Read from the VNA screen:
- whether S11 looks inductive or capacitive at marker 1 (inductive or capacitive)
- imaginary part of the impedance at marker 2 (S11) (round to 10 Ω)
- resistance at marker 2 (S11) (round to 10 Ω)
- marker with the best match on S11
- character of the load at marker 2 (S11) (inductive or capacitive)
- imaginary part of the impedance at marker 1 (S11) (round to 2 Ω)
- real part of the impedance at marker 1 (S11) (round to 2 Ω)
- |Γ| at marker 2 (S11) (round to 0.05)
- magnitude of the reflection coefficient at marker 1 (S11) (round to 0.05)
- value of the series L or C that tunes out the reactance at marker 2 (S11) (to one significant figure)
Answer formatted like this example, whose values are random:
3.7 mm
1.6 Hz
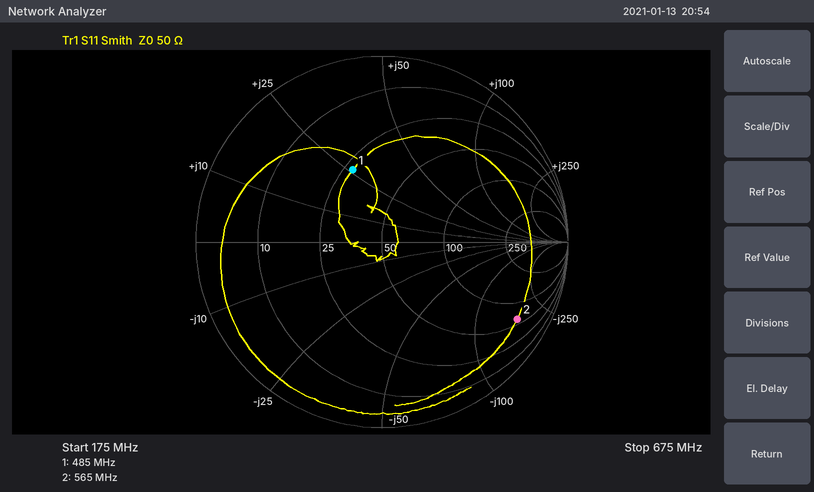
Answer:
inductive
-170 Ω
60 Ω
marker 1
capacitive
+26 Ω
28 Ω
0.85
0.40
50 nH
